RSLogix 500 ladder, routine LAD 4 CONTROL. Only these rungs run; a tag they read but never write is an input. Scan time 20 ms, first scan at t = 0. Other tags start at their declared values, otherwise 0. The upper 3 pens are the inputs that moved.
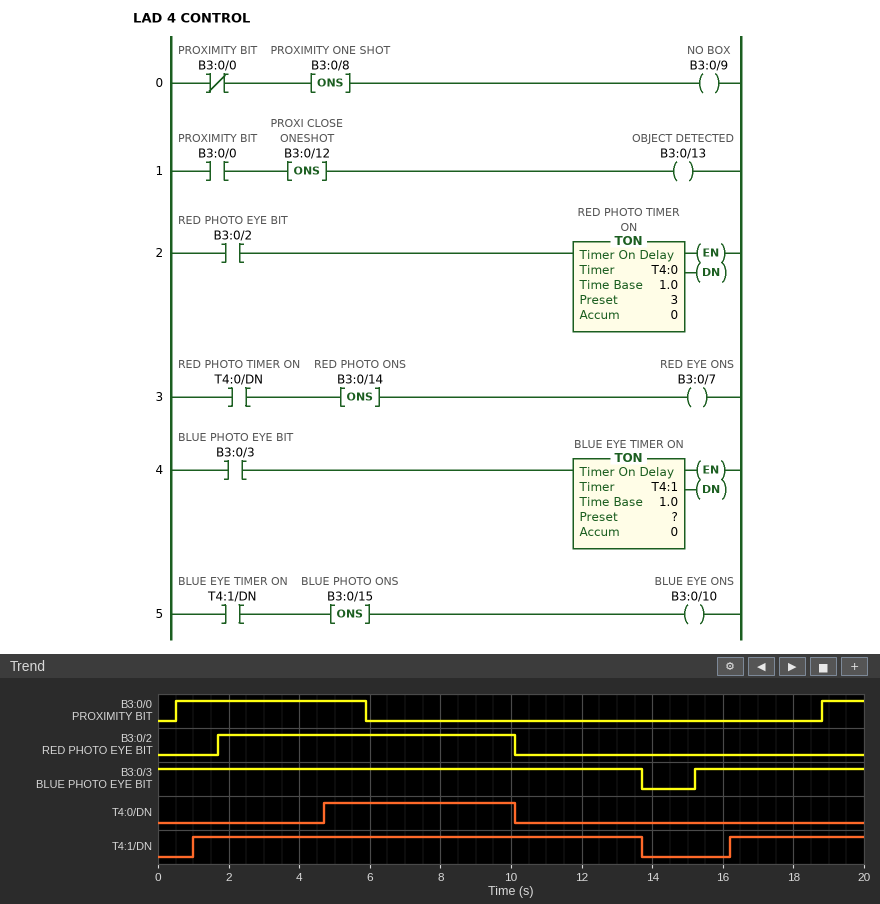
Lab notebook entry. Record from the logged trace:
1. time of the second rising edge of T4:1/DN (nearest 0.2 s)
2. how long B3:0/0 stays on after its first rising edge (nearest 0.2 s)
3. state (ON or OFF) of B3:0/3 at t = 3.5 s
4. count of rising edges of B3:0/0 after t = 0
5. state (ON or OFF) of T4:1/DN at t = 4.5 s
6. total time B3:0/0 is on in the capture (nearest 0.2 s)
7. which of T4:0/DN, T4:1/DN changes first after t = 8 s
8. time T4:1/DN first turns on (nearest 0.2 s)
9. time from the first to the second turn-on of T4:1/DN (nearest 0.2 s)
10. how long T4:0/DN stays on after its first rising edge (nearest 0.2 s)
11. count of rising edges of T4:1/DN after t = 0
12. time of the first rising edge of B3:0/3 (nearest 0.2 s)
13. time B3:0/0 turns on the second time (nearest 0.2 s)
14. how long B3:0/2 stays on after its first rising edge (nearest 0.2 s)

16.2 s
5.4 s
ON
2
ON
6.6 s
T4:0/DN
1.0 s
15.2 s
5.4 s
2
15.2 s
18.8 s
8.4 s
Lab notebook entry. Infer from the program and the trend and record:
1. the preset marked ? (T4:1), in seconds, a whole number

1 s
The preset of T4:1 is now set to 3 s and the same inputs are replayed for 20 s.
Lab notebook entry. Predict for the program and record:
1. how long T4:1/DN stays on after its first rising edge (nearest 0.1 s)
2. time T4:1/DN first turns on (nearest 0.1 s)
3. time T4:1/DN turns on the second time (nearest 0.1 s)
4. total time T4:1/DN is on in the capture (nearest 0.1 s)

10.7 s
3.0 s
18.2 s
12.5 s
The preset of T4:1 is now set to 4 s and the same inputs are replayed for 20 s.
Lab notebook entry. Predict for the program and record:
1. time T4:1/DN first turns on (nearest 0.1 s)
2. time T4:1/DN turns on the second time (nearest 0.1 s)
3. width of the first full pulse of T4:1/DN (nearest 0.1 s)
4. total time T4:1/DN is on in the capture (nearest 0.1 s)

4.0 s
19.2 s
9.7 s
10.5 s
